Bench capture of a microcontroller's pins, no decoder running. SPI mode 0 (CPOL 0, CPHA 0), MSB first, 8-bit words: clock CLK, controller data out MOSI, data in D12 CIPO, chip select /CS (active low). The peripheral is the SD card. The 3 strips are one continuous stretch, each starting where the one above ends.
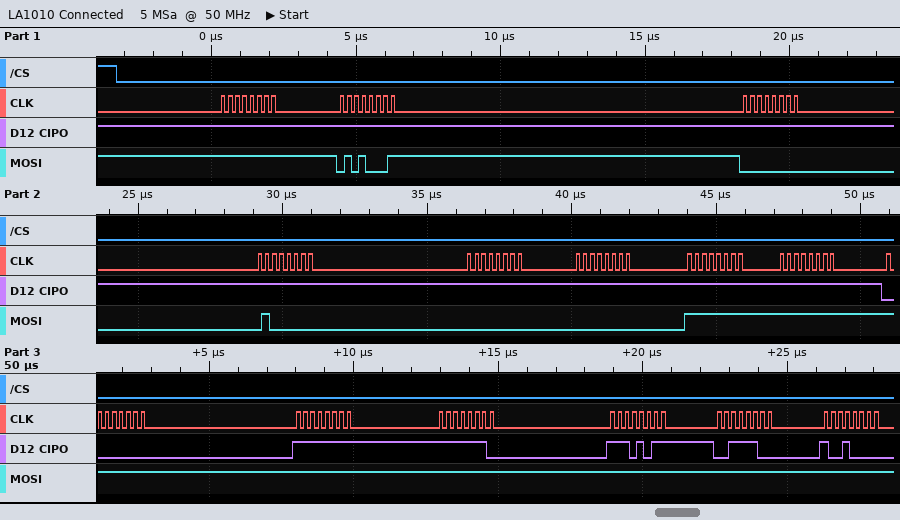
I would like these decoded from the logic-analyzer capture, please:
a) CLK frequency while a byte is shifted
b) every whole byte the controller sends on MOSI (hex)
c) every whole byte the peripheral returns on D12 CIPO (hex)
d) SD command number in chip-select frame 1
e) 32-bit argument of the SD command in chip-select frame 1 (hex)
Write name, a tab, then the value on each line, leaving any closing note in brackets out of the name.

CLK frequency while a byte is shifted	4 MHz
every whole byte the controller sends on MOSI	0xFF 0x51 0x00 0x40 0x00 0x00 0xFF 0xFF 0xFF 0xFF 0xFF 0xFF 0xFF 0xFF
every whole byte the peripheral returns on D12 CIPO	0xFF 0xFF 0xFF 0xFF 0xFF 0xFF 0xFF 0xFF 0x00 0xFF 0xFE 0xEB 0x3C 0x90
SD command number in chip-select frame 1	CMD17
32-bit argument of the SD command in chip-select frame 1	0x00400000
